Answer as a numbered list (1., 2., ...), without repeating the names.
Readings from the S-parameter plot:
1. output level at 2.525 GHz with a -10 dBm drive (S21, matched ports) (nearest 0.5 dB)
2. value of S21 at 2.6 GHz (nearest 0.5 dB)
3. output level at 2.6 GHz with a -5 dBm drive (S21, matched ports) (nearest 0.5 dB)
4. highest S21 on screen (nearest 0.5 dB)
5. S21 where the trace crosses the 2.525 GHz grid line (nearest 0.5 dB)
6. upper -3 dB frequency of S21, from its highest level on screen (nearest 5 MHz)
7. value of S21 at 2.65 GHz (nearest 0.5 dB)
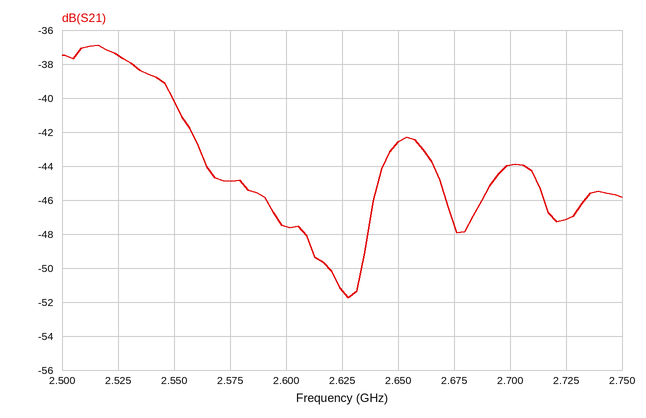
1. -47.5 dBm
2. -47.5 dB
3. -52.5 dBm
4. -37.0 dB
5. -37.5 dB
6. 2.550 GHz
7. -42.5 dB
